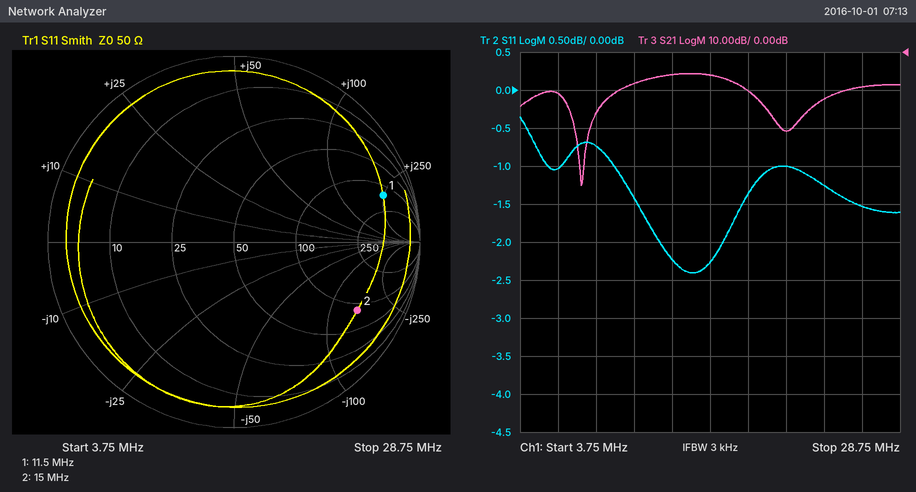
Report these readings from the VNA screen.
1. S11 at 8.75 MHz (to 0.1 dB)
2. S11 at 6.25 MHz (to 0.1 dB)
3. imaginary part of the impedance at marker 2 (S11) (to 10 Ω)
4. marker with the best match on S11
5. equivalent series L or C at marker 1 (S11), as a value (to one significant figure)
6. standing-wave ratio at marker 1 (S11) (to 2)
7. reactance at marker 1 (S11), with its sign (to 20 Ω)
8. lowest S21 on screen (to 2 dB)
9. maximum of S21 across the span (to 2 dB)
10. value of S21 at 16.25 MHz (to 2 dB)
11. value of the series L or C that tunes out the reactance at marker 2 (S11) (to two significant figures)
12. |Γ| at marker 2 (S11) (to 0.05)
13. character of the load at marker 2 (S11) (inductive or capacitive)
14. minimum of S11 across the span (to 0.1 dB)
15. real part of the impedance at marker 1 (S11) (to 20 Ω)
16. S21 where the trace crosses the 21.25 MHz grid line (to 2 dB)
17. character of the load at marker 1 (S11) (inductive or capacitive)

-0.7 dB
-1.0 dB
-150 Ω
marker 2
3 µH
12
+240 Ω
-36 dB
-6 dB
-6 dB
1.6 µH
0.75
capacitive
-2.4 dB
140 Ω
-20 dB
inductive
